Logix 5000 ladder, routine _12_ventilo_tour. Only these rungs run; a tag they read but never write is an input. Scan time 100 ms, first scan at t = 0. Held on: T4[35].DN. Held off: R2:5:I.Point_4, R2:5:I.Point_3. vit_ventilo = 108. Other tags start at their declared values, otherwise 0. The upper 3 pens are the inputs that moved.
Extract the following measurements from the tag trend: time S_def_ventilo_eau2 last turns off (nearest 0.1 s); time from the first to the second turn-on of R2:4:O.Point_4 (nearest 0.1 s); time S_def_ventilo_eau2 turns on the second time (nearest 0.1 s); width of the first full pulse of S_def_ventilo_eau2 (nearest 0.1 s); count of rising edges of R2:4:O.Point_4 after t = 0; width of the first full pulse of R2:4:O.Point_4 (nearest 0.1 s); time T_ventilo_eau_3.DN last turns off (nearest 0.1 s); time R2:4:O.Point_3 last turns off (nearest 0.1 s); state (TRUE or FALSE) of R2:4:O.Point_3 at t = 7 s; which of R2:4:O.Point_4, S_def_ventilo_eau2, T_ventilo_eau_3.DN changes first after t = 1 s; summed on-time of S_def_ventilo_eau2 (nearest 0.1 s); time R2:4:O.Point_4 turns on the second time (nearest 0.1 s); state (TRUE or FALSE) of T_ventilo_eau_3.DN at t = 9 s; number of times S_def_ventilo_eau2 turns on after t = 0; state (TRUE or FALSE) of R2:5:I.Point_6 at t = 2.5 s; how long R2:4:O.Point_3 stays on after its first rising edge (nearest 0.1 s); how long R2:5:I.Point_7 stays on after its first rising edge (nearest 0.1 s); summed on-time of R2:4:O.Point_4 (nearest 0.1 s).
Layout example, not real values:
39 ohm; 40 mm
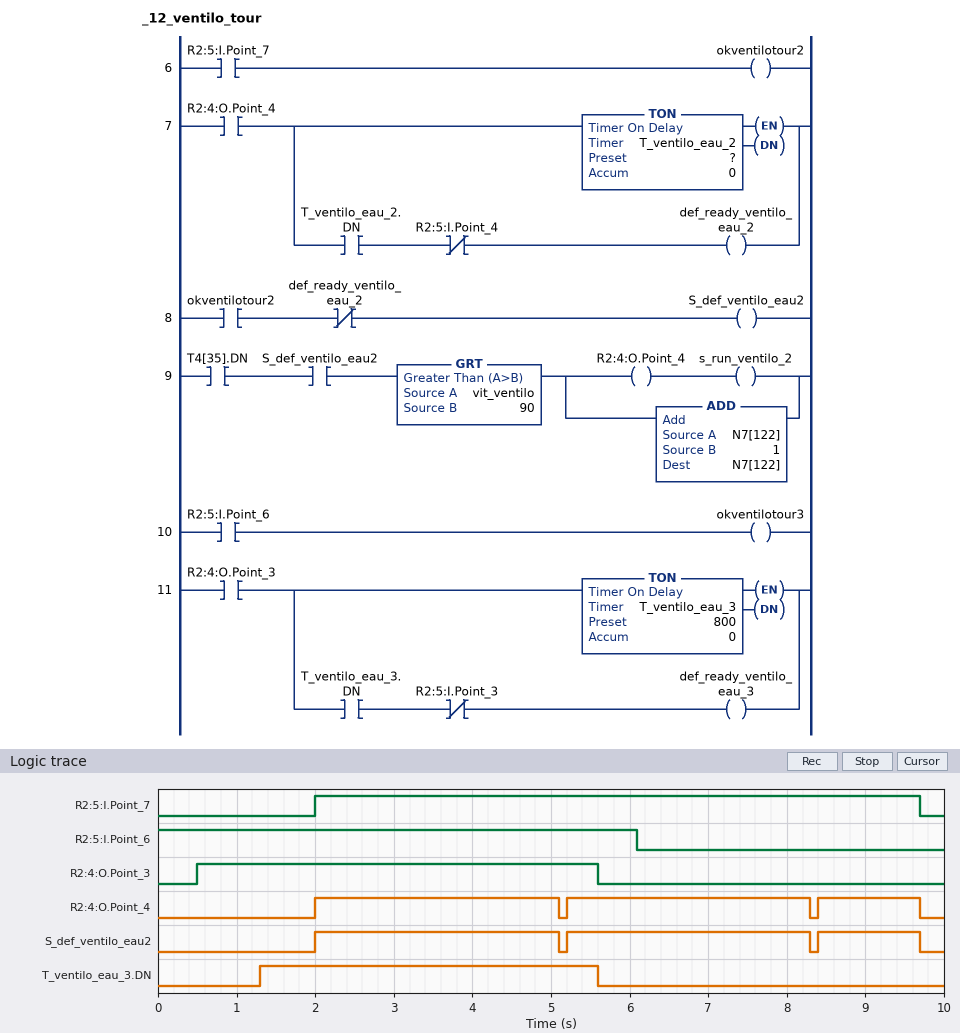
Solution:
9.7 s; 3.2 s; 5.2 s; 3.1 s; 3; 3.1 s; 5.6 s; 5.6 s; FALSE; T_ventilo_eau_3.DN; 7.5 s; 5.2 s; FALSE; 3; TRUE; 5.1 s; 7.7 s; 7.5 s
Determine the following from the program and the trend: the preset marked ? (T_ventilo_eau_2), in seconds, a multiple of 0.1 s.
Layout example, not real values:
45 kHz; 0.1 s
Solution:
3.0 s
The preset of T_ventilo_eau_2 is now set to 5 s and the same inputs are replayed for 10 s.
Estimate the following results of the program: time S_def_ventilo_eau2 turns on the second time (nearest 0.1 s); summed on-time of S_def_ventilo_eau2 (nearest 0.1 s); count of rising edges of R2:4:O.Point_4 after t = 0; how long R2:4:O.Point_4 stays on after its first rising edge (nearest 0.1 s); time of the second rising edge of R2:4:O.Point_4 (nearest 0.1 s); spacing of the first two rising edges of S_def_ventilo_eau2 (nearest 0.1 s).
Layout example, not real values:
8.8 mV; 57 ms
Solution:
7.2 s; 7.6 s; 2; 5.1 s; 7.2 s; 5.2 s
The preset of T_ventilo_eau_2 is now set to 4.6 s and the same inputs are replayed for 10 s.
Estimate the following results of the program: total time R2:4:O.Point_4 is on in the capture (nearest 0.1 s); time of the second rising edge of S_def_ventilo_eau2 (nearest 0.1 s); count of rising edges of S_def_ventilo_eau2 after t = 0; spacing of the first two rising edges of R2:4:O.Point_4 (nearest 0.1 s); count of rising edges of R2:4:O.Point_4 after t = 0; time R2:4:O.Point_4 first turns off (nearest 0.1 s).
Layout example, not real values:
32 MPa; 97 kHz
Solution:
7.6 s; 6.8 s; 2; 4.8 s; 2; 6.7 s
